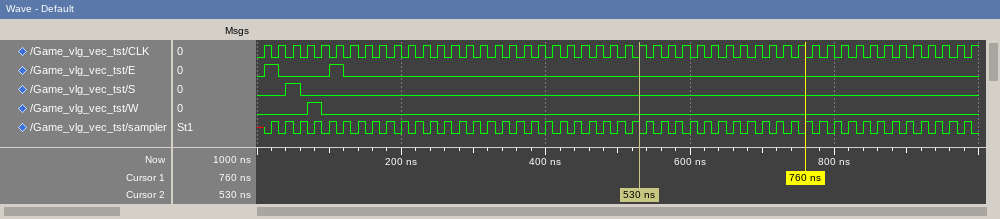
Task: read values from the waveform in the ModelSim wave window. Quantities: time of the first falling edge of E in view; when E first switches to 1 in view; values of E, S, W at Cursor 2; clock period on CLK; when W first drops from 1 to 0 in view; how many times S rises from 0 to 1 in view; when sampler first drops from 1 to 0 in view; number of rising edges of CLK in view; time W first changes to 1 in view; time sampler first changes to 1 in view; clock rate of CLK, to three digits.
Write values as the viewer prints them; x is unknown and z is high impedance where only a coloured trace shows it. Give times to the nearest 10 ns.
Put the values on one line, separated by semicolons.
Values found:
30 ns; 10 ns; E=0, S=0, W=0; 20 ns; 90 ns; 1; 30 ns; 50; 70 ns; 20 ns; 50.0 MHz
